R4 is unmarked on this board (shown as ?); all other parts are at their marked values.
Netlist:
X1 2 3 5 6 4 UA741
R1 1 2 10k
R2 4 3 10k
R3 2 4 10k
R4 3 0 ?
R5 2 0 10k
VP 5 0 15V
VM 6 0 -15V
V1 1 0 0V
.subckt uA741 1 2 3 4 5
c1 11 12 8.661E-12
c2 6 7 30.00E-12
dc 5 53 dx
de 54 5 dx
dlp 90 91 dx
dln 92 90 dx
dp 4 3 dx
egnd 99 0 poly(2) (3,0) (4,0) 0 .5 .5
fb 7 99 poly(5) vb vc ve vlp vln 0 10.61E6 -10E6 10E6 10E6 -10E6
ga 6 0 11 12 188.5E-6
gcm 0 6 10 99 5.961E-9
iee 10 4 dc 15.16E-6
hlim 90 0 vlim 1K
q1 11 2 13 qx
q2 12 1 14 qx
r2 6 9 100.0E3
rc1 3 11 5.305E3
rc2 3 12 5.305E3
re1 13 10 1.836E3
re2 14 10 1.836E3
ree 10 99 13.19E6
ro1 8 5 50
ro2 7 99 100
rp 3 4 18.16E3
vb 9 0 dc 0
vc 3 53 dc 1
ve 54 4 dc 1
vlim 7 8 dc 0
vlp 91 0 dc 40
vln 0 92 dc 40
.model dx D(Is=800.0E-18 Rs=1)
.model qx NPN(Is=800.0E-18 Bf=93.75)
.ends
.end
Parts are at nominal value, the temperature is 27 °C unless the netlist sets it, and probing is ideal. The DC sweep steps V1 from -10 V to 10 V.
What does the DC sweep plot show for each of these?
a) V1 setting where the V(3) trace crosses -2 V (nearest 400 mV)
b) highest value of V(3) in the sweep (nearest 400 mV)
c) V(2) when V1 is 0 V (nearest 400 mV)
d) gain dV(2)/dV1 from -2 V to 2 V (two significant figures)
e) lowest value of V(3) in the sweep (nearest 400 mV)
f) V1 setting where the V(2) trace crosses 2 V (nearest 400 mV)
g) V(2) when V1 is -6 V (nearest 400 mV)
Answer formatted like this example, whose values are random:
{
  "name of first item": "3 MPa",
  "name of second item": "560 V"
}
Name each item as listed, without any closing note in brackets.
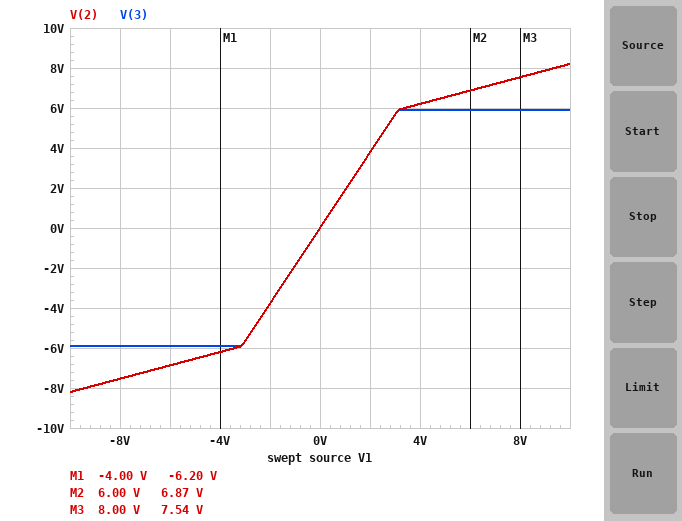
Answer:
{
  "V1 setting where the V(3) trace crosses -2 V": "-1.2 V",
  "highest value of V(3) in the sweep": "6.0 V",
  "V(2) when V1 is 0 V": "0 V",
  "gain dV(2)/dV1 from -2 V to 2 V": "1.9 V/V",
  "lowest value of V(3) in the sweep": "-6.0 V",
  "V1 setting where the V(2) trace crosses 2 V": "1.2 V",
  "V(2) when V1 is -6 V": "-6.8 V"
}
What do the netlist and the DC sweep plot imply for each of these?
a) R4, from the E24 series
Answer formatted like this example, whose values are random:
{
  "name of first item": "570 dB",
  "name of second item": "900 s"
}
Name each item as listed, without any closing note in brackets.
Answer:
{
  "R4, from the E24 series": "6.8 kΩ"
}
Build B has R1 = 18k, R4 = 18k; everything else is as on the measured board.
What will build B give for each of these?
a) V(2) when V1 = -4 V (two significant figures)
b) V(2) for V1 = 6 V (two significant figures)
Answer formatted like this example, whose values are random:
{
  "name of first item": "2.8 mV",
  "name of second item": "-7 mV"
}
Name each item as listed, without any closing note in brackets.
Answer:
{
  "V(2) when V1 = -4 V": "-2.2 V",
  "V(2) for V1 = 6 V": "3.3 V"
}
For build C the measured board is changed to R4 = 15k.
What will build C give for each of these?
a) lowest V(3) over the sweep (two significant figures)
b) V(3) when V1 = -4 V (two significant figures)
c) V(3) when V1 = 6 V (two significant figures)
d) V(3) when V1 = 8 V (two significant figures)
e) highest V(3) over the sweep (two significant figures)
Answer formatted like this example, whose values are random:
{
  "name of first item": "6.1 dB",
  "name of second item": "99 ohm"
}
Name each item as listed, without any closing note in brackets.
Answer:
{
  "lowest V(3) over the sweep": "-7.5 V",
  "V(3) when V1 = -4 V": "-3.0 V",
  "V(3) when V1 = 6 V": "4.5 V",
  "V(3) when V1 = 8 V": "6.0 V",
  "highest V(3) over the sweep": "7.5 V"
}
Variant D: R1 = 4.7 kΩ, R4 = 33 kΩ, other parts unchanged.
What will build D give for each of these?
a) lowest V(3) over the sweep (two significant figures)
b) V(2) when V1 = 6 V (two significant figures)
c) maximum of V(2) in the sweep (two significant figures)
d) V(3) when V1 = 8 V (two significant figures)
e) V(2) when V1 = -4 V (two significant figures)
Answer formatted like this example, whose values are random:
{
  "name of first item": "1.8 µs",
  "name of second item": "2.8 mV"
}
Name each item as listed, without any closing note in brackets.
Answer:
{
  "lowest V(3) over the sweep": "-7.5 V",
  "V(2) when V1 = 6 V": "4.5 V",
  "maximum of V(2) in the sweep": "7.5 V",
  "V(3) when V1 = 8 V": "6.0 V",
  "V(2) when V1 = -4 V": "-3.0 V"
}
